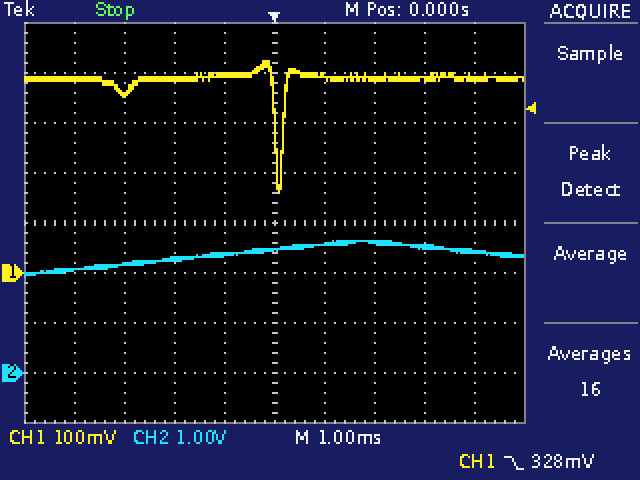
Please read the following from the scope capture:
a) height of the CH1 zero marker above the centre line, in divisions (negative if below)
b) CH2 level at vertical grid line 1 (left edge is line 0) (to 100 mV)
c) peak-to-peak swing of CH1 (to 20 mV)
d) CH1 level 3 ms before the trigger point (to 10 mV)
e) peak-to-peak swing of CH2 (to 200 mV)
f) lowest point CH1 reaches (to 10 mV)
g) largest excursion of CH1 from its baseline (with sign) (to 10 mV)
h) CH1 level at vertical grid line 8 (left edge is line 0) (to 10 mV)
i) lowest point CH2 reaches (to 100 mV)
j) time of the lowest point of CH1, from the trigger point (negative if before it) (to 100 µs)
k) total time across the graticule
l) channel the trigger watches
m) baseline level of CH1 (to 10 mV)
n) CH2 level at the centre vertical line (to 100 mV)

-1.0 div
2.1 V
260 mV
360 mV
800 mV
160 mV
-230 mV
390 mV
1.9 V
+100 µs
10 ms
CH1
390 mV
2.5 V
